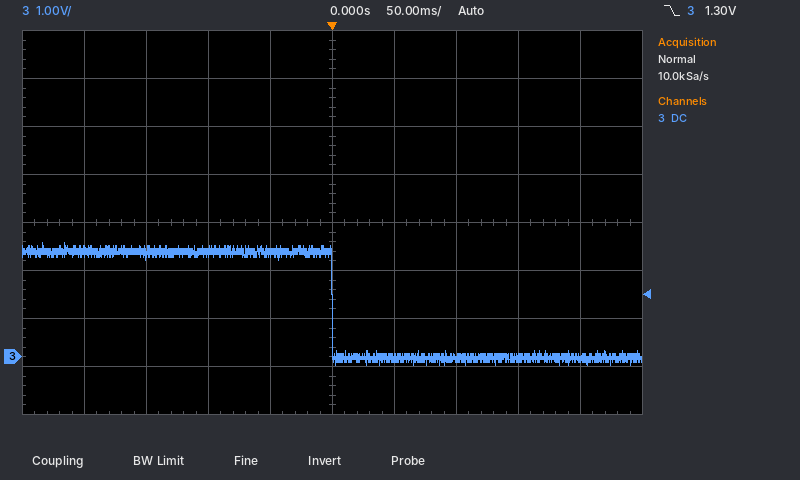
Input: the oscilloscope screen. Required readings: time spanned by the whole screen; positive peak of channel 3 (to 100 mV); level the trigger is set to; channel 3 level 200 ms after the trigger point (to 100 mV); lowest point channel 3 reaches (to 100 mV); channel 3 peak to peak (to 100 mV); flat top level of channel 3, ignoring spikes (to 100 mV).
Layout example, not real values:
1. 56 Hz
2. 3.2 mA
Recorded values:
1. 500 ms
2. 2.4 V
3. 1.30 V
4. 0.0 V
5. -200 mV
6. 2.6 V
7. 2.2 V
